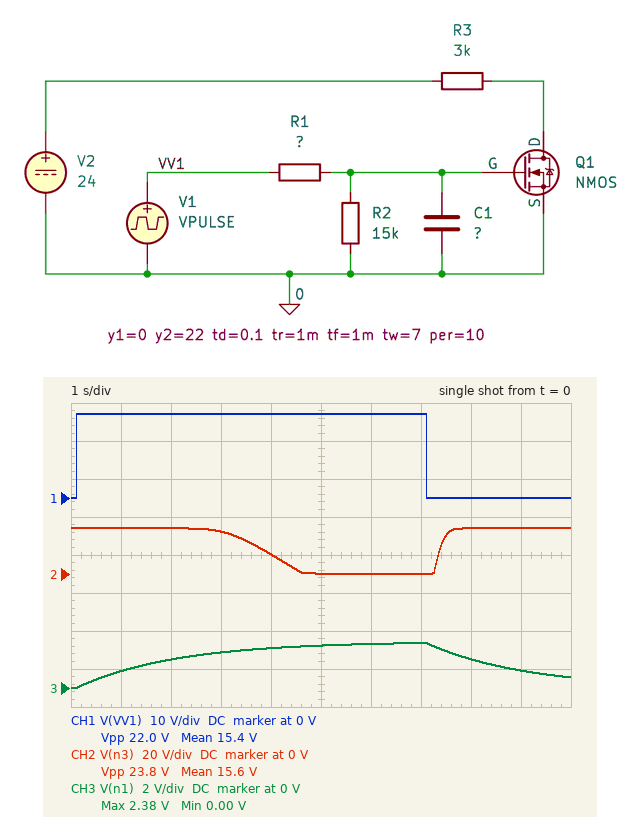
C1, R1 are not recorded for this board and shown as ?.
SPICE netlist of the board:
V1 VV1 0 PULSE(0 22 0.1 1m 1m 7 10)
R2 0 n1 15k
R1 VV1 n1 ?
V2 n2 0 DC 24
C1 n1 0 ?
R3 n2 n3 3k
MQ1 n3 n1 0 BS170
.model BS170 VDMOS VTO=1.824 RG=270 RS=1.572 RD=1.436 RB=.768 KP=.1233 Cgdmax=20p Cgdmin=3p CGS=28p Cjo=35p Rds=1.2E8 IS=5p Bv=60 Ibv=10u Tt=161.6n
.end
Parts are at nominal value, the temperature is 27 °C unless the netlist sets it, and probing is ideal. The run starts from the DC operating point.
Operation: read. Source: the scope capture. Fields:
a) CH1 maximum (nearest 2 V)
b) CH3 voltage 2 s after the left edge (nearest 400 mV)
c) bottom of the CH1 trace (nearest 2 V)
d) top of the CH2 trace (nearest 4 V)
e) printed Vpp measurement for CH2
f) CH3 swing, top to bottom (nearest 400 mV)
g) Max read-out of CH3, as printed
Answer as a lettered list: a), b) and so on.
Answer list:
a) 22 V
b) 1.6 V
c) 0 V
d) 24 V
e) 23.8 V
f) 2.4 V
g) 2.38 V
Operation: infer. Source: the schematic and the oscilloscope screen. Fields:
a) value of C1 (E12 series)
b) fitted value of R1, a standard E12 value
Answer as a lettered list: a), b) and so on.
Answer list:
a) 150 µF
b) 120 kΩ
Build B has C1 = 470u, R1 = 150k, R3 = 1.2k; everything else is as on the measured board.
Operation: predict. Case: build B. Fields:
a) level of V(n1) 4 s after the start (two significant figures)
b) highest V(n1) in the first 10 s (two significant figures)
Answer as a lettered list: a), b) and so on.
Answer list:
a) 910 mV
b) 1.3 V
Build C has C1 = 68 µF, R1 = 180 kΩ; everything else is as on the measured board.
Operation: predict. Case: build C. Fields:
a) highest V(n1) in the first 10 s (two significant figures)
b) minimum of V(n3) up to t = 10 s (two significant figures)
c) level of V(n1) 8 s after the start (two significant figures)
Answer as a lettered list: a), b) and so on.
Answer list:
a) 1.7 V
b) 24 V
c) 650 mV
